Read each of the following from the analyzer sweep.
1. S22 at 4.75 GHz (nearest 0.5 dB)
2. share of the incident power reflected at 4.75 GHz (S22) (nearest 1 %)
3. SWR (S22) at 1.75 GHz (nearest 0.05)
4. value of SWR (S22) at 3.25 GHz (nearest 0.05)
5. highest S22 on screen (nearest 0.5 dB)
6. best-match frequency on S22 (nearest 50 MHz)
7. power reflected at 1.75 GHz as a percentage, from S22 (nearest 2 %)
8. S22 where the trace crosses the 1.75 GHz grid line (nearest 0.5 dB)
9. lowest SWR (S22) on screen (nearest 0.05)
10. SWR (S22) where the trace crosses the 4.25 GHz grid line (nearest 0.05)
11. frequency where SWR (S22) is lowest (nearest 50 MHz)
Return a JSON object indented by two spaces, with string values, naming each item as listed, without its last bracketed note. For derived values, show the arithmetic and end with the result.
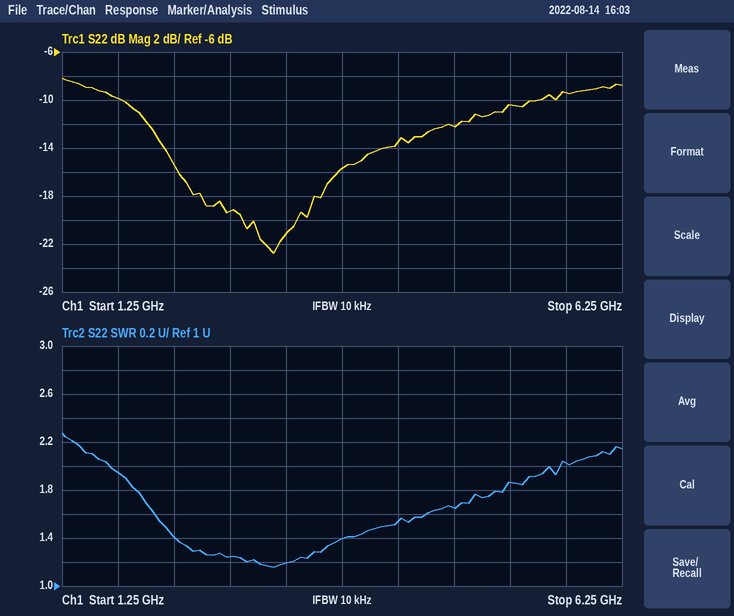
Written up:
{
  "S22 at 4.75 GHz": "-12.0 dB",
  "share of the incident power reflected at 4.75 GHz (S22)": "10^(-12/10) ≈ 6 %",
  "SWR (S22) at 1.75 GHz": "1.95",
  "value of SWR (S22) at 3.25 GHz": "1.20",
  "highest S22 on screen": "-8.0 dB",
  "best-match frequency on S22": "3.15 GHz",
  "power reflected at 1.75 GHz as a percentage, from S22": "10^(-10/10) ≈ 10 %",
  "S22 where the trace crosses the 1.75 GHz grid line": "-10.0 dB",
  "lowest SWR (S22) on screen": "1.15",
  "SWR (S22) where the trace crosses the 4.25 GHz grid line": "1.55",
  "frequency where SWR (S22) is lowest": "3.15 GHz"
}
